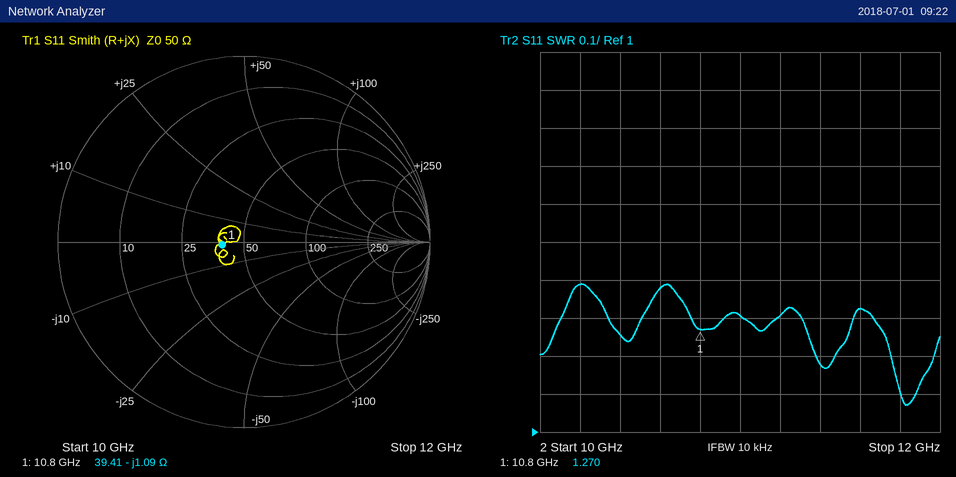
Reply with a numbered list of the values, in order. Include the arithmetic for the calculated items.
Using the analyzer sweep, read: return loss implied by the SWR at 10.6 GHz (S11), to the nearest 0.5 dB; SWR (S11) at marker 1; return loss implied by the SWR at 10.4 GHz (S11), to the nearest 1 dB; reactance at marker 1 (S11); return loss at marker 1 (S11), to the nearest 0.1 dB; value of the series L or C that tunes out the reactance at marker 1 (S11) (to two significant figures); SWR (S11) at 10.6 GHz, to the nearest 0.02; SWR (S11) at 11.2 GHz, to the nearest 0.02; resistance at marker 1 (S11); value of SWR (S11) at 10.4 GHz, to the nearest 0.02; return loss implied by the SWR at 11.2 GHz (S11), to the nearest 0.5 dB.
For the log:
1. −20 log10((1.38 − 1)/(1.38 + 1)) ≈ 15.9 dB, so 16.0 dB to the nearest 0.5 dB
2. 1.270
3. −20 log10((1.26 − 1)/(1.26 + 1)) ≈ 19 dB
4. -1.09 Ω
5. 18.5 dB
6. L = 1.09 Ω/(2π × 10.8 GHz) ≈ 16 pH
7. 1.38
8. 1.30
9. 39.41 Ω
10. 1.26
11. −20 log10((1.3 − 1)/(1.3 + 1)) ≈ 17.7 dB, so 17.5 dB to the nearest 0.5 dB
